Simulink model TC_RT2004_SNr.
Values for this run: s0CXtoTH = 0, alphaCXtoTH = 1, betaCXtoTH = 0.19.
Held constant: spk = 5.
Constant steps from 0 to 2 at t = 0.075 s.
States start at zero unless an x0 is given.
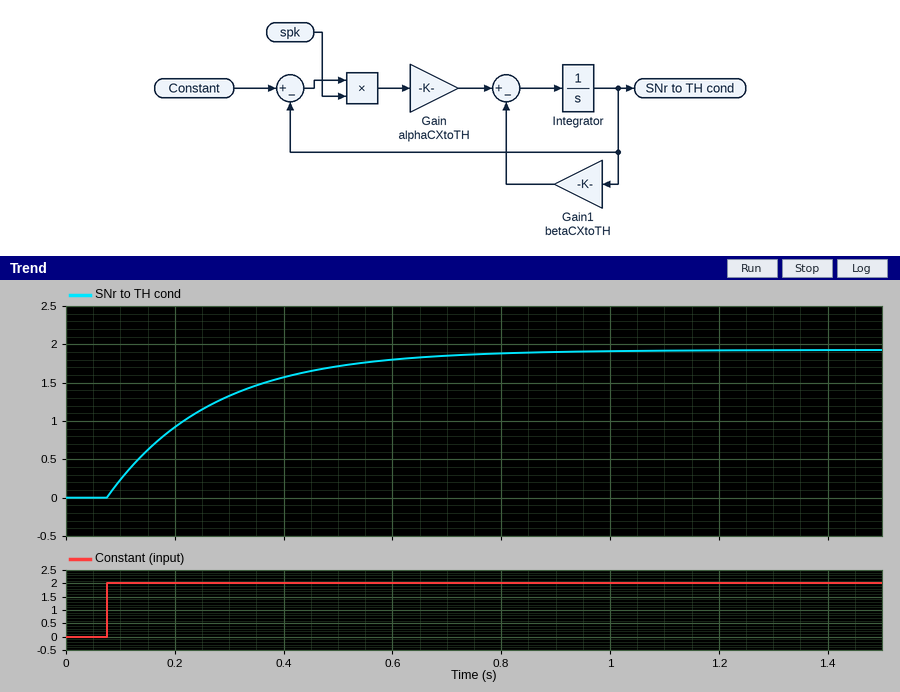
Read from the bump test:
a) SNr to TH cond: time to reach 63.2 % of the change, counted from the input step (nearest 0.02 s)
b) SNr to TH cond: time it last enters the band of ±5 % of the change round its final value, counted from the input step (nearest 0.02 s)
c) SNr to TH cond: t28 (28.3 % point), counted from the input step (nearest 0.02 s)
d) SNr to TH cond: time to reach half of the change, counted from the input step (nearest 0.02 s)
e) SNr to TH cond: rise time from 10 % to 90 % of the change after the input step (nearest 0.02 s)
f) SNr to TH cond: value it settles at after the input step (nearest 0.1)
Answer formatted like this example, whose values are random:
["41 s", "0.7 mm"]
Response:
["0.20 s", "0.58 s", "0.06 s", "0.14 s", "0.42 s", "1.9"]
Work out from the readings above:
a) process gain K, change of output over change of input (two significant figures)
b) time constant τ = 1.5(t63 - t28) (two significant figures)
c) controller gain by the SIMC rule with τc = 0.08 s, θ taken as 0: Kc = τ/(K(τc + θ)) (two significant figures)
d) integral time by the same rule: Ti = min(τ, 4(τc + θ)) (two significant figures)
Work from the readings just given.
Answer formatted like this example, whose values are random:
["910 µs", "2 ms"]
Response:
["0.95", "0.21 s", "2.8", "0.21 s"]
